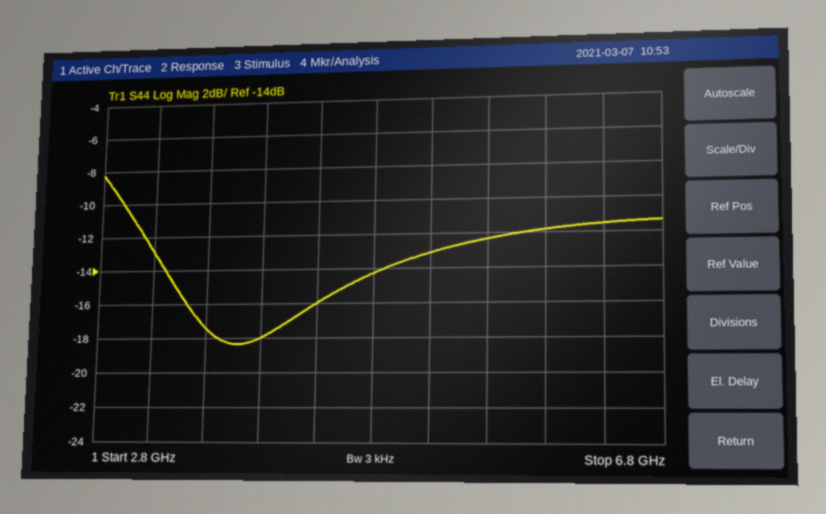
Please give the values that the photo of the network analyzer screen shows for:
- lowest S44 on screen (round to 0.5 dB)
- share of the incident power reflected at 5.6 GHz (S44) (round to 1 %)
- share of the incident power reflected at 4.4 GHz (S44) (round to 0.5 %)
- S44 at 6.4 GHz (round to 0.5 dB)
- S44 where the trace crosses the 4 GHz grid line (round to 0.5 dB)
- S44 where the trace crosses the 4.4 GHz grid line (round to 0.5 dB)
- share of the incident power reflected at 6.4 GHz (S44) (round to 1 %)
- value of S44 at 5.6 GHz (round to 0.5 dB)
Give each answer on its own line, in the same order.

-18.5 dB
6 %
2.5 %
-11.5 dB
-18.0 dB
-16.0 dB
7 %
-12.5 dB
